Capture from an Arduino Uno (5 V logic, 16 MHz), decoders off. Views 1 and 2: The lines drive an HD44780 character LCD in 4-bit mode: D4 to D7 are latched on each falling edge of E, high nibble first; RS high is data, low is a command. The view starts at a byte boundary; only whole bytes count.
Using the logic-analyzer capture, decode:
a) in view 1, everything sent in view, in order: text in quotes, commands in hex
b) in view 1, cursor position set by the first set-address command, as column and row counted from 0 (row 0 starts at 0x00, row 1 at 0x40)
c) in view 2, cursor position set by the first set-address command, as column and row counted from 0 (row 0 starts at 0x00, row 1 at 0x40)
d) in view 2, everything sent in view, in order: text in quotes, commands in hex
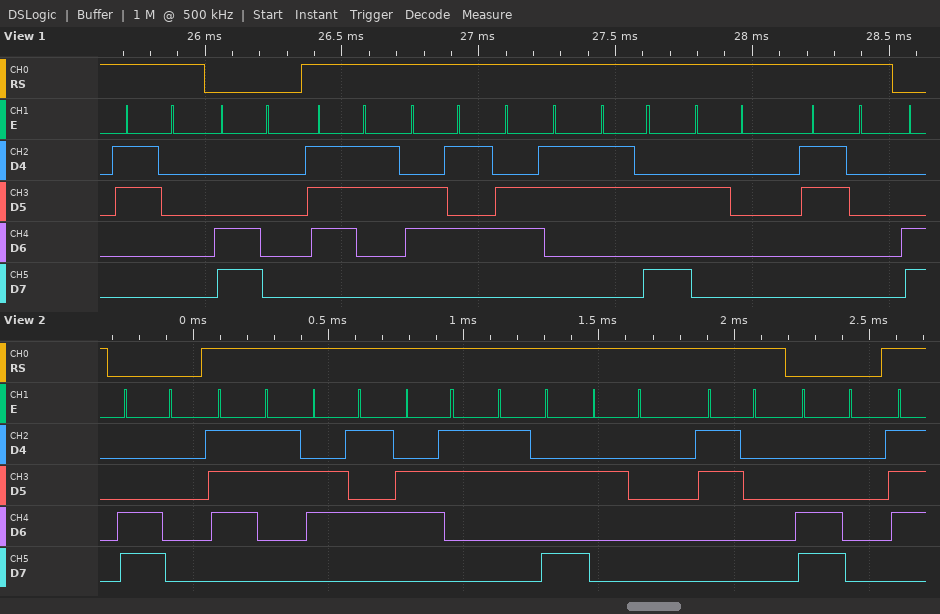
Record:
"0" 0xC0 "sec: 0"
column 0, row 1
column 0, row 1
0xC0 "sec: 0" 0xC0
